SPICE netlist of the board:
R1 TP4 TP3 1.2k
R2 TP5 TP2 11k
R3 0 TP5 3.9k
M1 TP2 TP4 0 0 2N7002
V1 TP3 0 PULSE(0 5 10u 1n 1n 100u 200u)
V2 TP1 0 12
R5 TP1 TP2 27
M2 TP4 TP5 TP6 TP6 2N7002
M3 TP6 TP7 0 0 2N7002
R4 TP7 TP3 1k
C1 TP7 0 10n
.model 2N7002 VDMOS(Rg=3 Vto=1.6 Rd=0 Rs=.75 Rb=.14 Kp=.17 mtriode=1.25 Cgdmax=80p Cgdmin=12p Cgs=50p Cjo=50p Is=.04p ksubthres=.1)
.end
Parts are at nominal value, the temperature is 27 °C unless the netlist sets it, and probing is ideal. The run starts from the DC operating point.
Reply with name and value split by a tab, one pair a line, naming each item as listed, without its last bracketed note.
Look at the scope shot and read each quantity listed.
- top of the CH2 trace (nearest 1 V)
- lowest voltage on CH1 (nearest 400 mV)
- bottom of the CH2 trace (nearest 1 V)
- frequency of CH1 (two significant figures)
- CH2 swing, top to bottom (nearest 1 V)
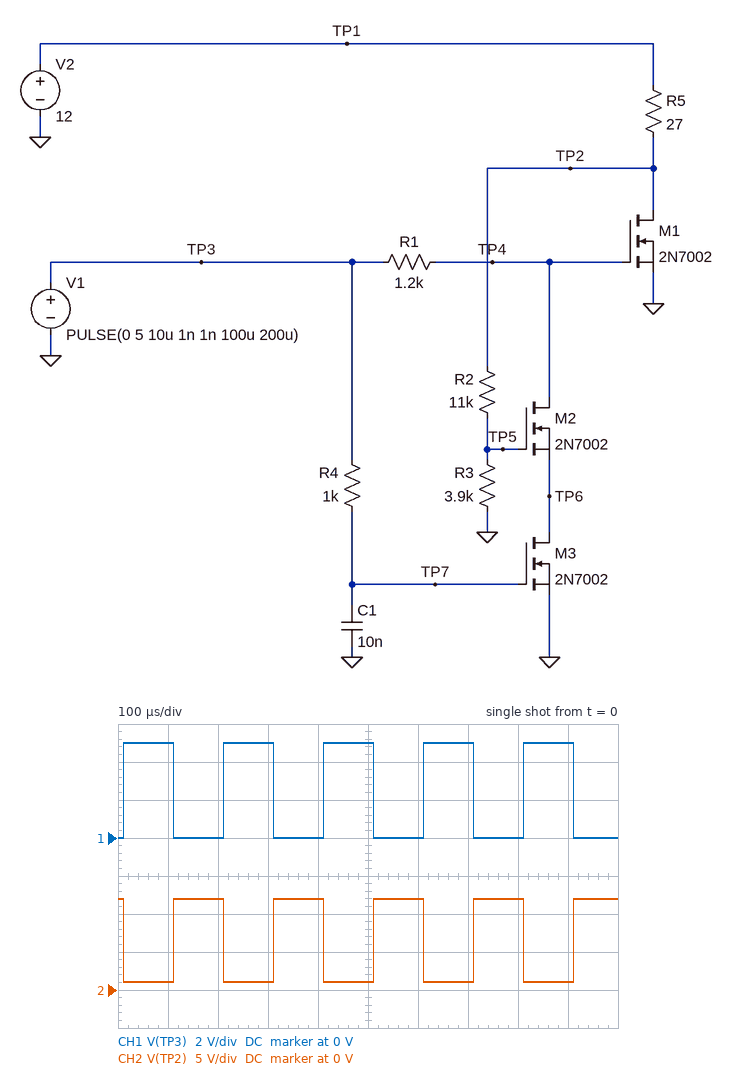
top of the CH2 trace	12 V
lowest voltage on CH1	0 V
bottom of the CH2 trace	1 V
frequency of CH1	5.0 kHz
CH2 swing, top to bottom	11 V
